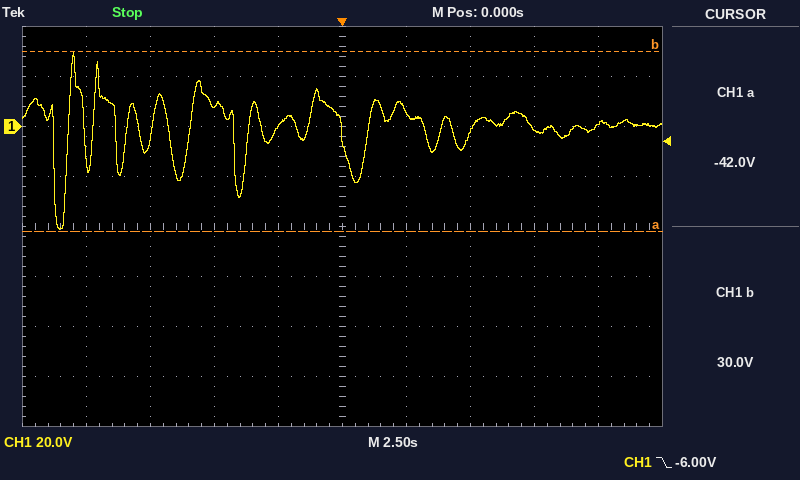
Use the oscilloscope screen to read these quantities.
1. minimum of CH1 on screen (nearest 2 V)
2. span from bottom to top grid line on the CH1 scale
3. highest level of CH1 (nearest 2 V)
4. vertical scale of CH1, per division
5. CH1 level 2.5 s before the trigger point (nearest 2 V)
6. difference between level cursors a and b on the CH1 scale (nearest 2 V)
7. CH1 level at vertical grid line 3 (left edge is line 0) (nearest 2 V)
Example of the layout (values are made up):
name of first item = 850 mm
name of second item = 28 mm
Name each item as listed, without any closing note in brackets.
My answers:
minimum of CH1 on screen = -42 V
span from bottom to top grid line on the CH1 scale = 160 V
highest level of CH1 = 30 V
vertical scale of CH1, per division = 20 V
CH1 level 2.5 s before the trigger point = 0 V
difference between level cursors a and b on the CH1 scale = 72 V
CH1 level at vertical grid line 3 (left edge is line 0) = 8 V
